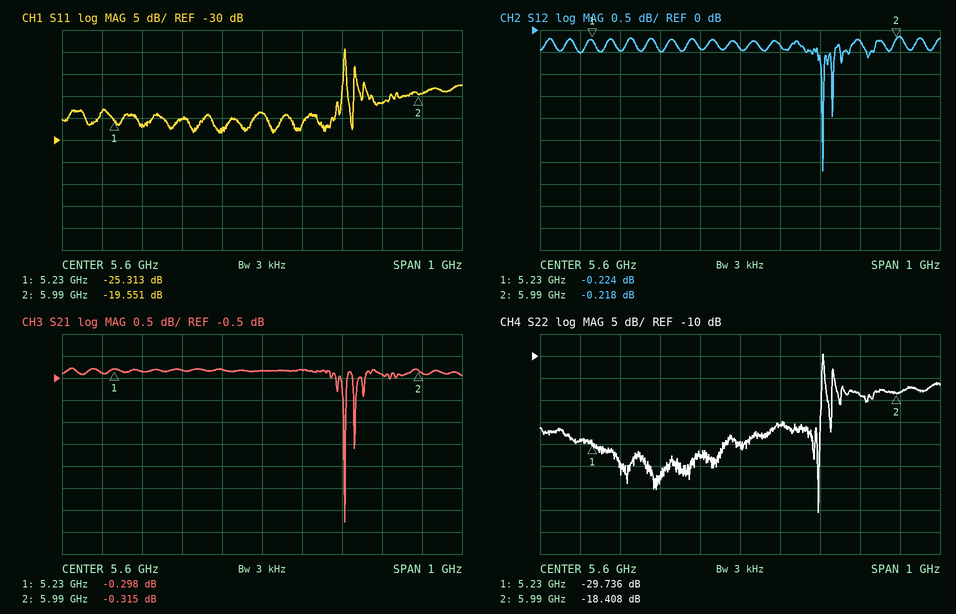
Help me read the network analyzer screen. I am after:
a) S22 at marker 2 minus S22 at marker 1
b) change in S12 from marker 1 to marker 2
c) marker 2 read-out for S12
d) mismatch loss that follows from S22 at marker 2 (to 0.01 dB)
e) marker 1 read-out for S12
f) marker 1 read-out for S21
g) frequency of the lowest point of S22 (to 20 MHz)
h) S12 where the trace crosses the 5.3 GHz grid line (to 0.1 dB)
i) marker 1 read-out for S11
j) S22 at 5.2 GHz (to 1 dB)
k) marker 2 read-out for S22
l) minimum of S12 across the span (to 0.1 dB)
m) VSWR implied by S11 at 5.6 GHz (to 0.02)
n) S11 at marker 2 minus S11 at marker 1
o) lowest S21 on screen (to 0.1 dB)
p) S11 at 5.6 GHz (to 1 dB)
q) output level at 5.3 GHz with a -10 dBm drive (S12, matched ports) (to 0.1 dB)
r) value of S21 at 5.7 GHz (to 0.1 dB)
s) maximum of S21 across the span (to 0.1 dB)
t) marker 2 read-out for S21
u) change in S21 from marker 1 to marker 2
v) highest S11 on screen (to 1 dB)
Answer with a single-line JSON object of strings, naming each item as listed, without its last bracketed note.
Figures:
{"S22 at marker 2 minus S22 at marker 1": "11.328 dB", "change in S12 from marker 1 to marker 2": "0.006 dB", "marker 2 read-out for S12": "-0.218 dB", "mismatch loss that follows from S22 at marker 2": "0.06 dB", "marker 1 read-out for S12": "-0.224 dB", "marker 1 read-out for S21": "-0.298 dB", "frequency of the lowest point of S22": "5.80 GHz", "S12 where the trace crosses the 5.3 GHz grid line": "-0.5 dB", "marker 1 read-out for S11": "-25.313 dB", "S22 at 5.2 GHz": "-29 dB", "marker 2 read-out for S22": "-18.408 dB", "minimum of S12 across the span": "-3.2 dB", "VSWR implied by S11 at 5.6 GHz": "1.14", "S11 at marker 2 minus S11 at marker 1": "5.762 dB", "lowest S21 on screen": "-3.8 dB", "S11 at 5.6 GHz": "-24 dB", "output level at 5.3 GHz with a -10 dBm drive (S12, matched ports)": "-10.5 dBm", "value of S21 at 5.7 GHz": "-0.3 dB", "maximum of S21 across the span": "-0.3 dB", "marker 2 read-out for S21": "-0.315 dB", "change in S21 from marker 1 to marker 2": "-0.017 dB", "highest S11 on screen": "-9 dB"}
